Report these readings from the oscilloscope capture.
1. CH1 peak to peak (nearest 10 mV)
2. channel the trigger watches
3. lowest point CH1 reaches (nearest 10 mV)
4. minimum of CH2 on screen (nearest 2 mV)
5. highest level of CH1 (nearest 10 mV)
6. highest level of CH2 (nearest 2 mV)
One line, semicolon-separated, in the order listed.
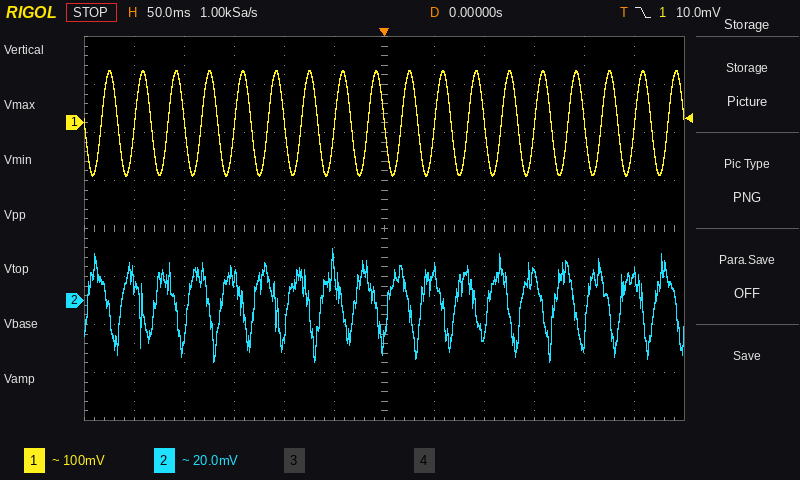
220 mV; CH1; -110 mV; -26 mV; 110 mV; 22 mV
